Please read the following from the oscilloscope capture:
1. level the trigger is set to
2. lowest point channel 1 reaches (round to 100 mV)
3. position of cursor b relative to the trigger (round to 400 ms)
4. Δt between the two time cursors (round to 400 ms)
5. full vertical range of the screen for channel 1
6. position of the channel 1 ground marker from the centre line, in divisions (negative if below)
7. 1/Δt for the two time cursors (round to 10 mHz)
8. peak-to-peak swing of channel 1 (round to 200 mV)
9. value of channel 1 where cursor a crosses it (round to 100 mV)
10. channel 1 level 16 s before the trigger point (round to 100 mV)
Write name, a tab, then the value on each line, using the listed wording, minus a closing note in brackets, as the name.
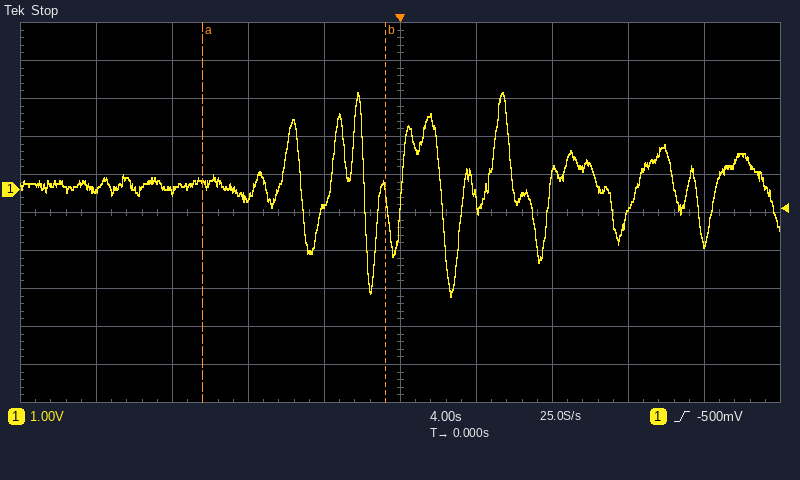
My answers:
level the trigger is set to	-500 mV
lowest point channel 1 reaches	-2.8 V
position of cursor b relative to the trigger	-800 ms
Δt between the two time cursors	9.6 s
full vertical range of the screen for channel 1	10 V
position of the channel 1 ground marker from the centre line, in divisions	+0.6 div
1/Δt for the two time cursors	100 mHz
peak-to-peak swing of channel 1	5.4 V
value of channel 1 where cursor a crosses it	200 mV
channel 1 level 16 s before the trigger point	0.0 V
